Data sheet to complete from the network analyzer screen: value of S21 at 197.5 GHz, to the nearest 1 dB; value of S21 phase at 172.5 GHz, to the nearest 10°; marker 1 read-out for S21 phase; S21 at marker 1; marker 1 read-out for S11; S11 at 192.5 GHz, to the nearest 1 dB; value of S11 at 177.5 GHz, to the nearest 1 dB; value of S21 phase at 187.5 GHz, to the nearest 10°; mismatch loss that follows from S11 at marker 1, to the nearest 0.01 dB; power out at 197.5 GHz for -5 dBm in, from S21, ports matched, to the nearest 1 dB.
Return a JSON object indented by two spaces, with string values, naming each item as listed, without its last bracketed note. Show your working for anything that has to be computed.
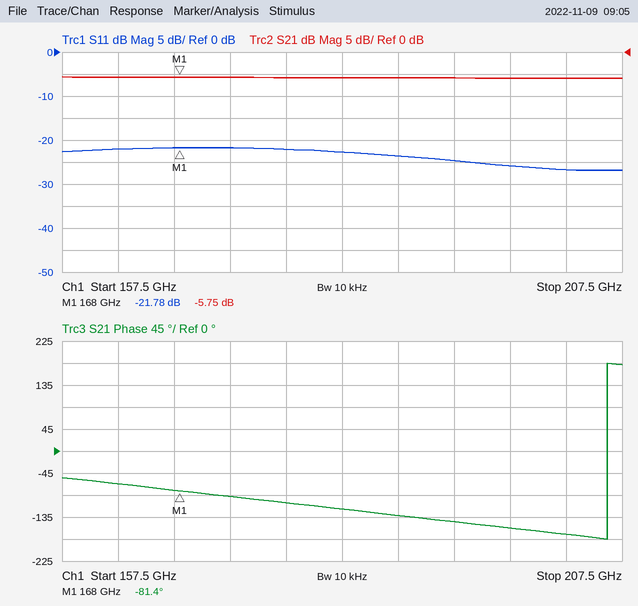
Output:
{
  "value of S21 at 197.5 GHz, to the nearest 1 dB": "-6 dB",
  "value of S21 phase at 172.5 GHz, to the nearest 10°": "-90°",
  "marker 1 read-out for S21 phase": "-81.4°",
  "S21 at marker 1": "-5.75 dB",
  "marker 1 read-out for S11": "-21.78 dB",
  "S11 at 192.5 GHz, to the nearest 1 dB": "-25 dB",
  "value of S11 at 177.5 GHz, to the nearest 1 dB": "-22 dB",
  "value of S21 phase at 187.5 GHz, to the nearest 10°": "-130°",
  "mismatch loss that follows from S11 at marker 1, to the nearest 0.01 dB": "−10 log10(1 − 10^(-21.78/10)) ≈ 0.03 dB",
  "power out at 197.5 GHz for -5 dBm in, from S21, ports matched, to the nearest 1 dB": "-5 dBm + (-6 dB) = -11 dBm"
}
